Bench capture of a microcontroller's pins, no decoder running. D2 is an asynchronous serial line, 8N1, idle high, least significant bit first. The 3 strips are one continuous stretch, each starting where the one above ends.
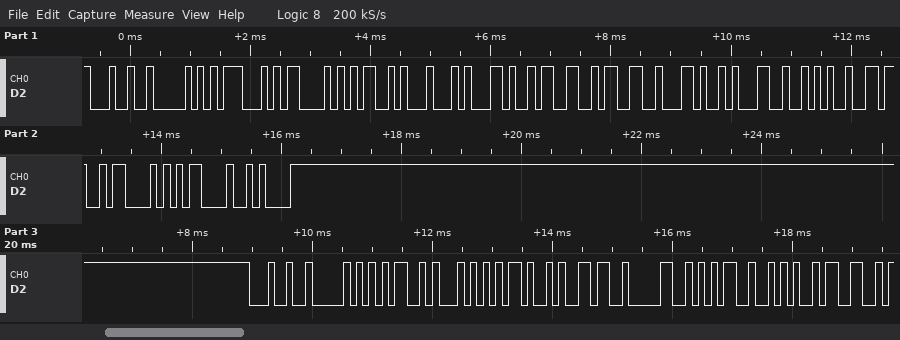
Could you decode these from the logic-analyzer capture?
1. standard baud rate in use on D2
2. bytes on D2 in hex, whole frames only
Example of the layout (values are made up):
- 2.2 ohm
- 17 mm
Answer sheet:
- 9600 baud
- 0x24 0x50 0x47 0x43 0x4D 0x44 0x2C 0x33 0x33 0x2C 0x31 0x2A 0x36 0x43 0x0D 0x0A 0x24 0x50 0x4D 0x54 0x4B 0x36 0x30 0x35 0x2A 0x33
